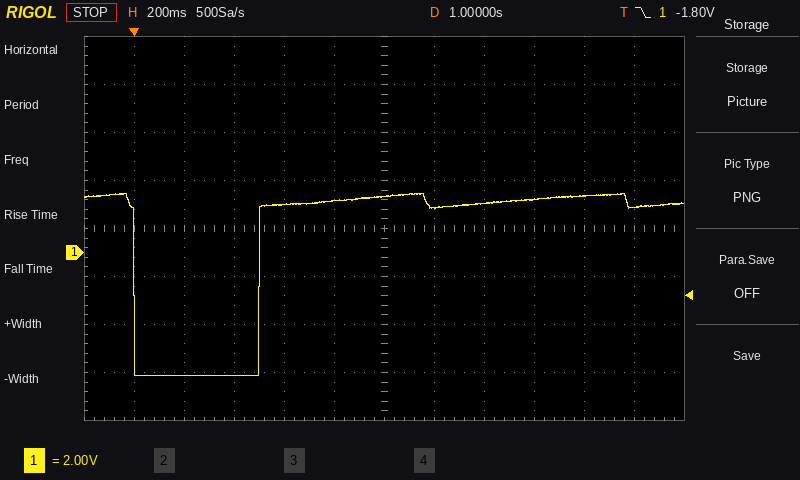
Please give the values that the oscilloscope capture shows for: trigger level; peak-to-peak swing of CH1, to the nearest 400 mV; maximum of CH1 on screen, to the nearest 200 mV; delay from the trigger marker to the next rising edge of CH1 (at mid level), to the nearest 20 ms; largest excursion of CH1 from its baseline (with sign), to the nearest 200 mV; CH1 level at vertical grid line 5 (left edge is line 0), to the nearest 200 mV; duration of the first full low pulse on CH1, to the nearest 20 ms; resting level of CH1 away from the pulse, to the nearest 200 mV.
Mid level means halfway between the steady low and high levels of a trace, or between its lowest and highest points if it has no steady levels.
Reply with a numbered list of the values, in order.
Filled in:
1. -1.80 V
2. 7.6 V
3. 2.4 V
4. 500 ms
5. -7.2 V
6. 2.2 V
7. 500 ms
8. 2.0 V
